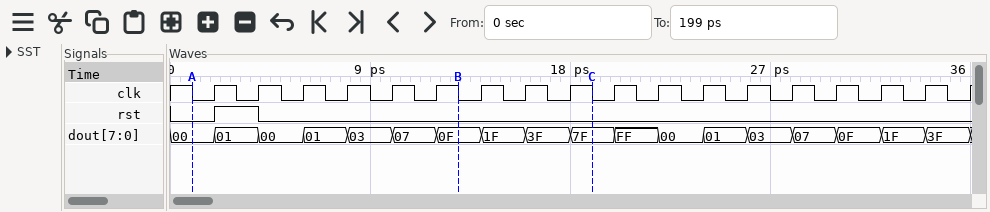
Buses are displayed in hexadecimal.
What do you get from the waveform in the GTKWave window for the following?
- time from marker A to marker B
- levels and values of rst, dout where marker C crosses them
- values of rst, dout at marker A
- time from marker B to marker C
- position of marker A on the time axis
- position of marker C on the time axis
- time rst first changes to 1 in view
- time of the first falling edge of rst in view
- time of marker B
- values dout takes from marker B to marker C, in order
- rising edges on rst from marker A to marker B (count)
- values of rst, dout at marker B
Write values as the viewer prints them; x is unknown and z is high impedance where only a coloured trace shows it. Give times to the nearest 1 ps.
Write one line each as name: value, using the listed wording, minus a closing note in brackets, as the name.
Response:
time from marker A to marker B: 12 ps
levels and values of rst, dout where marker C crosses them: rst=0, dout=7F
values of rst, dout at marker A: rst=0, dout=00
time from marker B to marker C: 6 ps
position of marker A on the time axis: 1 ps
position of marker C on the time axis: 19 ps
time rst first changes to 1 in view: 2 ps
time of the first falling edge of rst in view: 4 ps
time of marker B: 13 ps
values dout takes from marker B to marker C, in order: 0F, 1F, 3F, 7F
rising edges on rst from marker A to marker B: 1
values of rst, dout at marker B: rst=0, dout=0F
